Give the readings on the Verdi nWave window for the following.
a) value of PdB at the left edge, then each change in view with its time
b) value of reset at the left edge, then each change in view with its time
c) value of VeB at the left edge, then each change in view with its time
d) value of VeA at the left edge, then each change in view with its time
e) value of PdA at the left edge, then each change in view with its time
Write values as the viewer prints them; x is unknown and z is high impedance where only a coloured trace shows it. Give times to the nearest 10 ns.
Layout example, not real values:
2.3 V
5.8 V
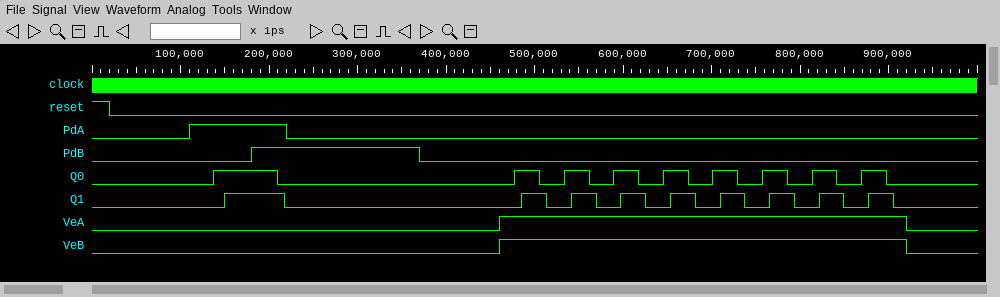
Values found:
0, 1 at 180 ns, 0 at 370 ns
1, 0 at 20 ns
0, 1 at 460 ns, 0 at 920 ns
0, 1 at 460 ns, 0 at 920 ns
0, 1 at 110 ns, 0 at 220 ns
